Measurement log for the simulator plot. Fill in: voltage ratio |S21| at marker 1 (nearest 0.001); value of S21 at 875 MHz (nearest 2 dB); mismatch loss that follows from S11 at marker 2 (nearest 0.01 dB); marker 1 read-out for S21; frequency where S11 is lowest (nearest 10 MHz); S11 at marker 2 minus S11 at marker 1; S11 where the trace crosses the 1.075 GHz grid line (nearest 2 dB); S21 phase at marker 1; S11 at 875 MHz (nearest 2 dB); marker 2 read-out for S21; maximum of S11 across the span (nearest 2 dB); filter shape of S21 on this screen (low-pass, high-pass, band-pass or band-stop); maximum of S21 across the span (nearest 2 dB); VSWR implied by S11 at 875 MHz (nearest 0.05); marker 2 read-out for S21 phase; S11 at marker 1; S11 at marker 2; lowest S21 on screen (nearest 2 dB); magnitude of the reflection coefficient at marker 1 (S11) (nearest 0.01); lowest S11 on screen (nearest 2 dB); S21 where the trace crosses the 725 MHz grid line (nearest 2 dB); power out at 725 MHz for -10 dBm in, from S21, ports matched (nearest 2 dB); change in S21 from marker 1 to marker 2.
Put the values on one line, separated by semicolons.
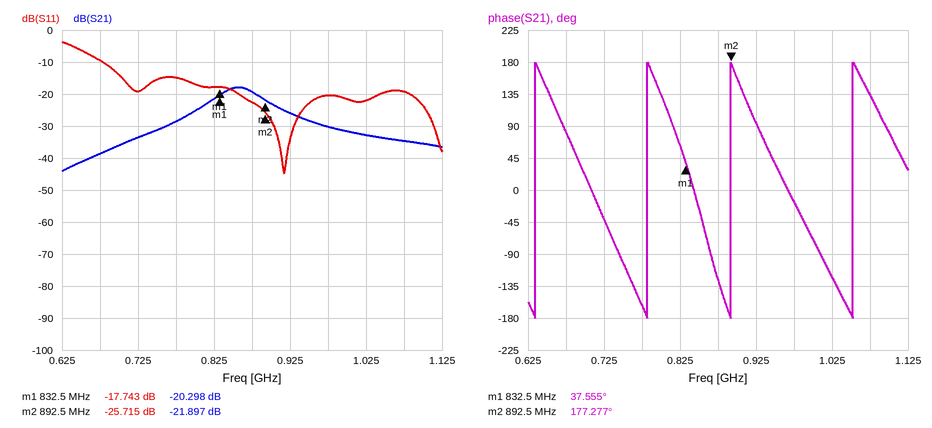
0.097; -20 dB; 0.01 dB; -20.298 dB; 920 MHz; -7.972 dB; -20 dB; 37.555°; -22 dB; -21.897 dB; -4 dB; band-pass; -18 dB; 1.15; 177.277°; -17.743 dB; -25.715 dB; -44 dB; 0.13; -44 dB; -34 dB; -44 dBm; -1.599 dB
